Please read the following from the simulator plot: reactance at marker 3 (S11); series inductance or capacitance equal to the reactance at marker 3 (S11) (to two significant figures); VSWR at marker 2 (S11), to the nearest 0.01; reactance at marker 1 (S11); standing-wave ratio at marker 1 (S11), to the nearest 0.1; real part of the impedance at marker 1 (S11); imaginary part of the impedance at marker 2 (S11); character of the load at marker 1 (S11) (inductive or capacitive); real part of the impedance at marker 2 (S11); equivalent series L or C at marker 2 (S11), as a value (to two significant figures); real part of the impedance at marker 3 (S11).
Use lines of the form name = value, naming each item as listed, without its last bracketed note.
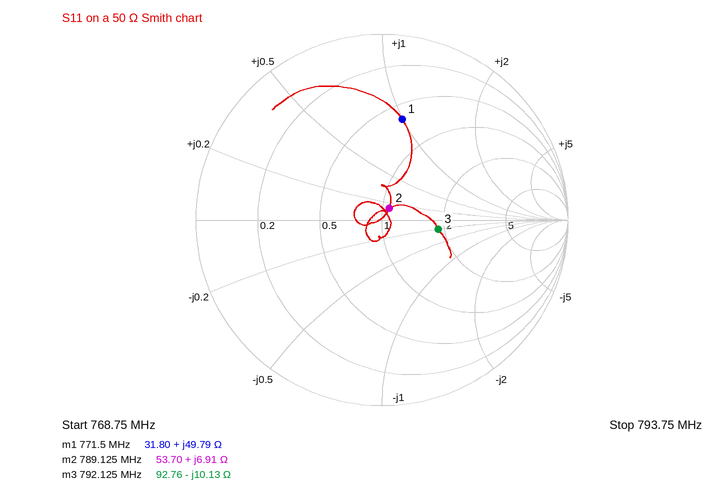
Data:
reactance at marker 3 = -10.13 Ω
series inductance or capacitance equal to the reactance at marker 3 (S11) = 20 pF
VSWR at marker 2 (S11), to the nearest 0.01 = 1.16
reactance at marker 1 = +49.79 Ω
standing-wave ratio at marker 1 (S11), to the nearest 0.1 = 3.5
real part of the impedance at marker 1 = 31.80 Ω
imaginary part of the impedance at marker 2 = +6.91 Ω
character of the load at marker 1 (S11) = inductive
real part of the impedance at marker 2 = 53.70 Ω
equivalent series L or C at marker 2 (S11), as a value = 1.4 nH
real part of the impedance at marker 3 = 92.76 Ω
